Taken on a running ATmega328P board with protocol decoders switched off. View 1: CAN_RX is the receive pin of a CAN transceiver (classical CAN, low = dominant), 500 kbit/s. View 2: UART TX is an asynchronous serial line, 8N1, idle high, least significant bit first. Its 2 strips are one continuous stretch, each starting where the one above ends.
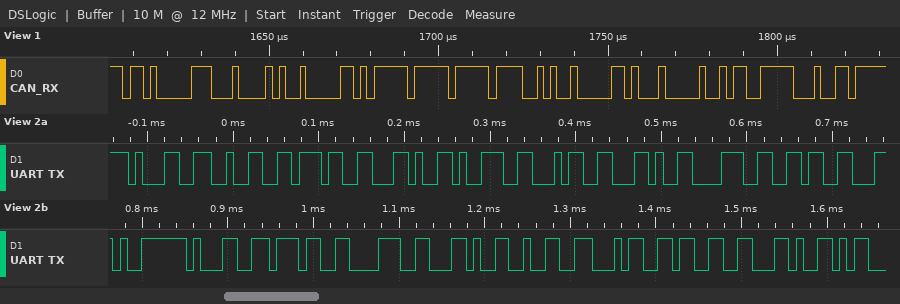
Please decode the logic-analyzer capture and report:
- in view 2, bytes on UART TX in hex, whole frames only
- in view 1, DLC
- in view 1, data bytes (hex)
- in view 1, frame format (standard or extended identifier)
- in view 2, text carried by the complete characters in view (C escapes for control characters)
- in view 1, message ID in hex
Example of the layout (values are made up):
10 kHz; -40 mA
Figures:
31 32 37 2C 39 34 2C 38 36 2C 31 37 38 2C 32 34 33 2C; 8; 52 0A FF FF E5 20 A2 02; standard; "127,94,86,178,243,"; 0x683
